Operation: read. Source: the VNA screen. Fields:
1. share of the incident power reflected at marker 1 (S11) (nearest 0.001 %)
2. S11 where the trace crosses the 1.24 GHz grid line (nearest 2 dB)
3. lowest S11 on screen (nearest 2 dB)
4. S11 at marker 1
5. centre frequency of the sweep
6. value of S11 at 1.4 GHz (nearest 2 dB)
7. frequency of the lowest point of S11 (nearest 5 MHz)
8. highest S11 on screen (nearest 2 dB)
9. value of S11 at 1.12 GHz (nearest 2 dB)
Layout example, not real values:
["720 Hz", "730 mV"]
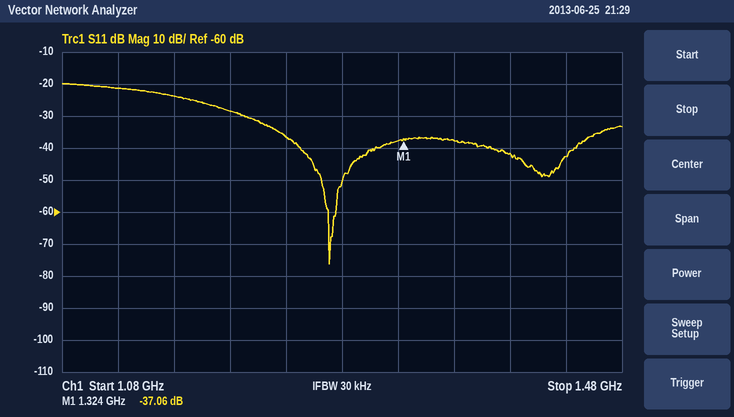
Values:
["0.020 %", "-36 dB", "-76 dB", "-37.06 dB", "1.28 GHz", "-42 dB", "1.270 GHz", "-20 dB", "-22 dB"]
